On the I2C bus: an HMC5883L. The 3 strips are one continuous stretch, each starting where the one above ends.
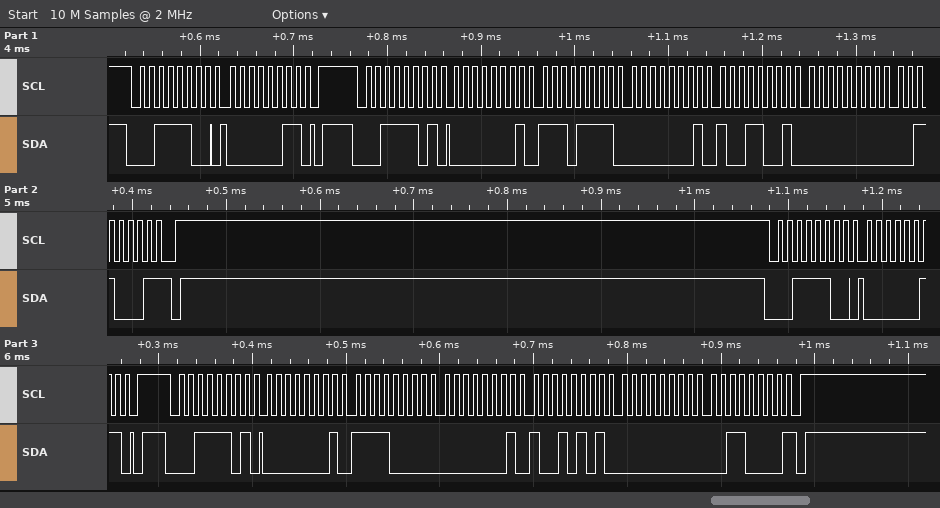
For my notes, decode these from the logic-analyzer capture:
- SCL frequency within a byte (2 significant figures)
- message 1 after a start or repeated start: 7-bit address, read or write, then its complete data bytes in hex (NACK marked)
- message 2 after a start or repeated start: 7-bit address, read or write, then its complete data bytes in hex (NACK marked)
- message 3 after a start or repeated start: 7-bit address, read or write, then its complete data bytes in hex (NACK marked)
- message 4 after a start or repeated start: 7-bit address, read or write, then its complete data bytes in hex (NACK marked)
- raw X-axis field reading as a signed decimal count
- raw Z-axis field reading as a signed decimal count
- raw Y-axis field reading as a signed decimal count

100 kHz
0x1E write: 03
0x1E read: 01 EF 01 99 00 31 NACK
0x1E write: 03
0x1E read: 01 F0 01 95 00 30 NACK
495
409
49
